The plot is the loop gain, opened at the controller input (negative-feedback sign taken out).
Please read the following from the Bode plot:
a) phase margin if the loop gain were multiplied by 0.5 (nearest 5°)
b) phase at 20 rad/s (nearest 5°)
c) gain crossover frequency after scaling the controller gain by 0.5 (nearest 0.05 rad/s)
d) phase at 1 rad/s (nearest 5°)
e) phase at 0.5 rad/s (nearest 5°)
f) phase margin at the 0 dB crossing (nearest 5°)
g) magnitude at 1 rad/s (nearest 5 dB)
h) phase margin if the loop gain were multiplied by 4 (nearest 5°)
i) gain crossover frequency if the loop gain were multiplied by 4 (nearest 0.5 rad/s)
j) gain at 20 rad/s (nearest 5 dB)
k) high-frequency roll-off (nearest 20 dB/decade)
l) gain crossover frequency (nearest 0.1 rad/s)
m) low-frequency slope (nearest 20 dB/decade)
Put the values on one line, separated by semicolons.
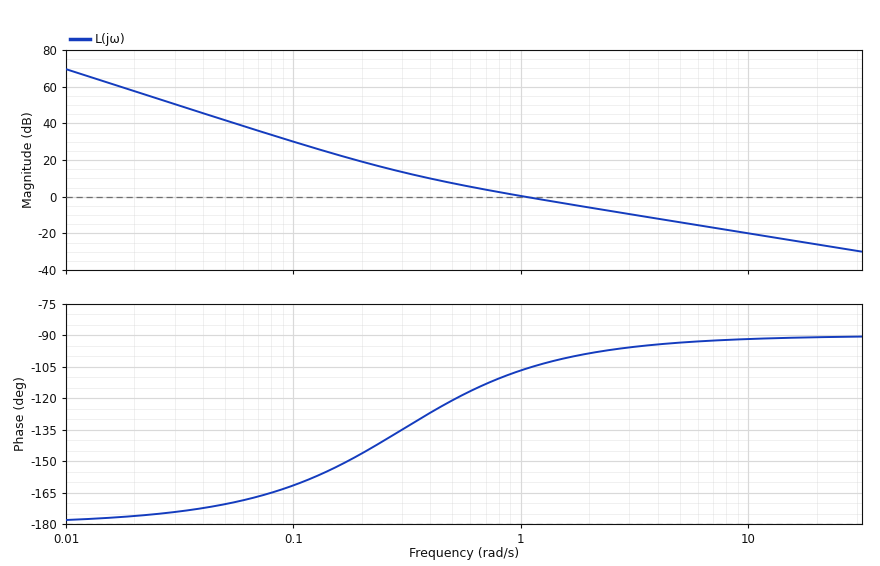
60°; -90°; 0.55 rad/s; -105°; -120°; 75°; 0 dB; 85°; 4.0 rad/s; -25 dB; -20 dB/decade; 1.0 rad/s; -40 dB/decade
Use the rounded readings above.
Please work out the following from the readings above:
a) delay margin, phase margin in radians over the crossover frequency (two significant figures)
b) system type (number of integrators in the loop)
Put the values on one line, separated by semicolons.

1.3 s; 2
